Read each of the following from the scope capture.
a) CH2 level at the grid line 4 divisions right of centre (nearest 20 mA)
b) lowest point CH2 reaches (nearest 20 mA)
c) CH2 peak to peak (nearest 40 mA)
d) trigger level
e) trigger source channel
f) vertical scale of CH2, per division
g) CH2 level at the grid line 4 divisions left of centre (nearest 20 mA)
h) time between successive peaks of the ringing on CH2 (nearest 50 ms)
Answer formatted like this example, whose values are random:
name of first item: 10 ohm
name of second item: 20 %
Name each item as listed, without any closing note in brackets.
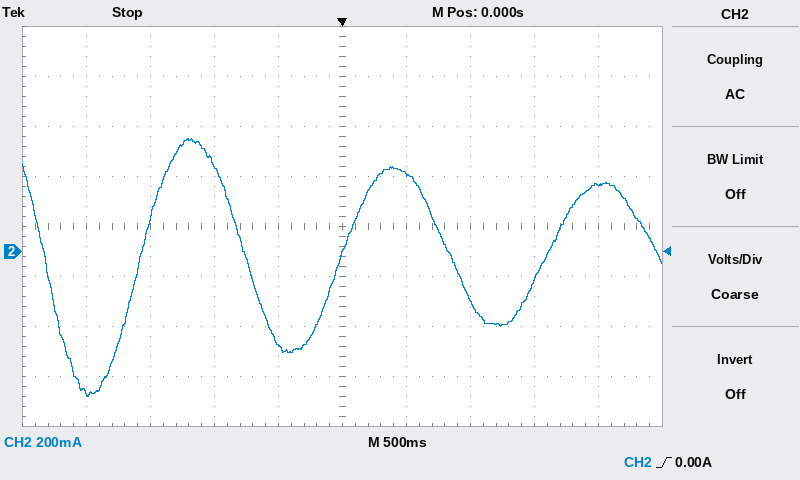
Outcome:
CH2 level at the grid line 4 divisions right of centre: 260 mA
lowest point CH2 reaches: -580 mA
CH2 peak to peak: 1.04 A
trigger level: 0.00 A
trigger source channel: CH2
vertical scale of CH2, per division: 200 mA
CH2 level at the grid line 4 divisions left of centre: -560 mA
time between successive peaks of the ringing on CH2: 1.65 s
